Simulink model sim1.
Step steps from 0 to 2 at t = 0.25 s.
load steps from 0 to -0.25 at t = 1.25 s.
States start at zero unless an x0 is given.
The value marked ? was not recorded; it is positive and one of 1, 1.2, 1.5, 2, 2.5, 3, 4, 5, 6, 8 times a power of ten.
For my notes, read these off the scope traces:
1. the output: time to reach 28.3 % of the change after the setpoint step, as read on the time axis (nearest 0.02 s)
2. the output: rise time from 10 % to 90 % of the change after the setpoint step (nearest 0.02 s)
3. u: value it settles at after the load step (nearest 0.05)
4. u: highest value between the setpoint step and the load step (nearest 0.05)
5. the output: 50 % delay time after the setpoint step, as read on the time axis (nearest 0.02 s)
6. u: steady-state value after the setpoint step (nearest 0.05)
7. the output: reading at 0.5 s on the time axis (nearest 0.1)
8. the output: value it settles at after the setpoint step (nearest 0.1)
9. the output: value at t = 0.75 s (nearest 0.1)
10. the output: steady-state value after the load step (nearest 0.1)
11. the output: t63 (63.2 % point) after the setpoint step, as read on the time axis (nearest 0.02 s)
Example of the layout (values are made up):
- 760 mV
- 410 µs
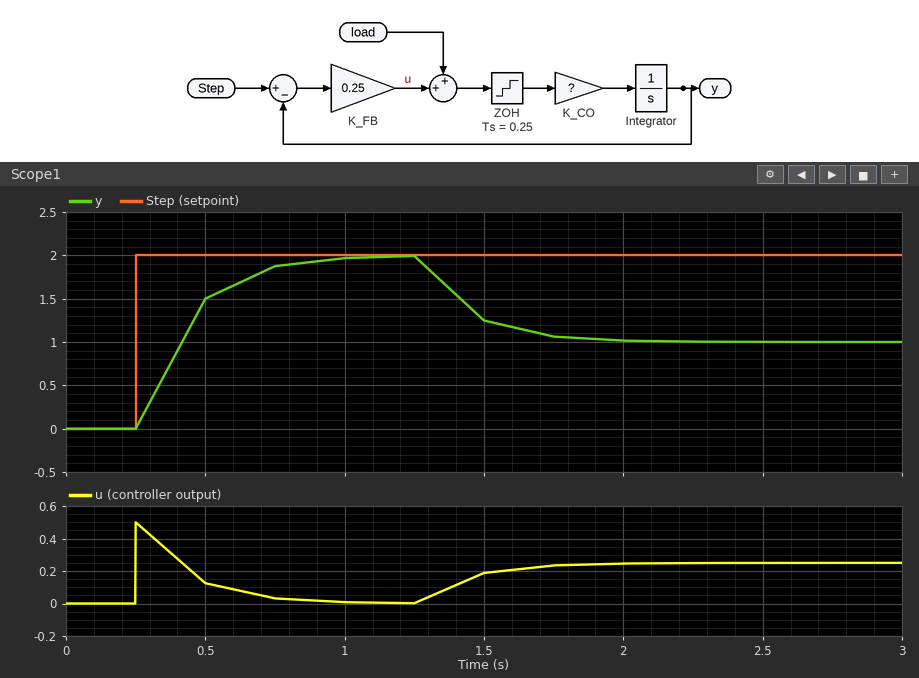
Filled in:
- 0.34 s
- 0.42 s
- 0.25
- 0.50
- 0.42 s
- 0.00
- 1.5
- 2.0
- 1.9
- 1.0
- 0.46 s
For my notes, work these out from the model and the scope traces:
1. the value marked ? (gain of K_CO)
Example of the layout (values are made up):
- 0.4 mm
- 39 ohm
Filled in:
- 12
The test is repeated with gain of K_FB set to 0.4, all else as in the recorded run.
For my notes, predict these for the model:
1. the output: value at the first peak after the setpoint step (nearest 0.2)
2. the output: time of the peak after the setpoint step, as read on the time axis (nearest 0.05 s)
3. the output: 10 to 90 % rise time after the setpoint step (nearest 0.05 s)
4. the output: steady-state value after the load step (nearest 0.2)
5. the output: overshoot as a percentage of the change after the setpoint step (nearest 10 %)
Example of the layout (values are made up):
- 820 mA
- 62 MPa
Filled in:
- 2.4
- 0.50 s
- 0.15 s
- 1.4
- 20 %
